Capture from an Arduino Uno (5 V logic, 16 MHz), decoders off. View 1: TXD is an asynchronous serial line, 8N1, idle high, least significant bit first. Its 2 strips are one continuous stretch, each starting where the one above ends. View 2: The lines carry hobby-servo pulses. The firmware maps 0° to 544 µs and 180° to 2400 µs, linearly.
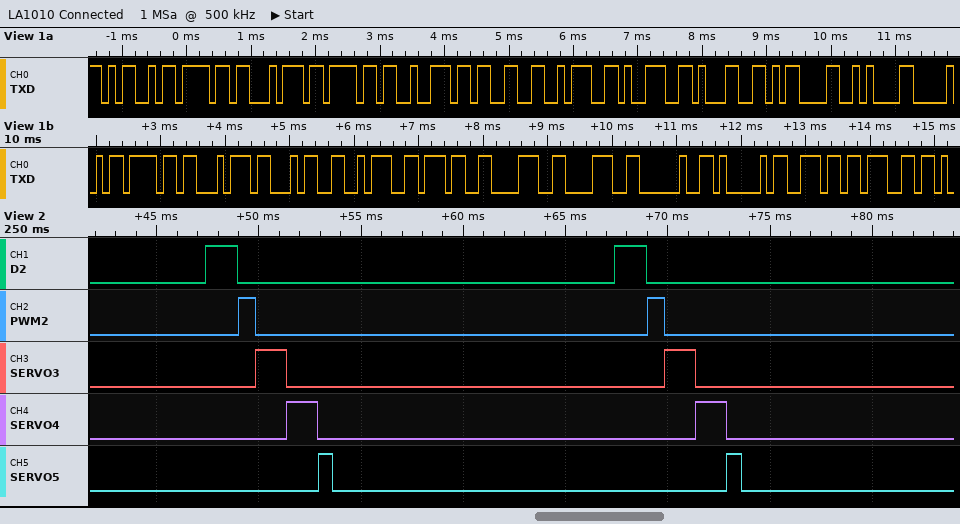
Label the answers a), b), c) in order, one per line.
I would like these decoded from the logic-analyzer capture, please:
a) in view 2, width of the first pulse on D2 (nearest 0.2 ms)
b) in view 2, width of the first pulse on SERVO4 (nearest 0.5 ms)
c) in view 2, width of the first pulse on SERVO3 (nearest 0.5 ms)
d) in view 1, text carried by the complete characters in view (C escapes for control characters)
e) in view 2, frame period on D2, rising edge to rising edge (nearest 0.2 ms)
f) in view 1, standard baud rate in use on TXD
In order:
a) 1.6 ms
b) 1.5 ms
c) 1.5 ms
d) "Motor3:91\r\nPot4:788 Ang"
e) 20.0 ms
f) 9600 baud
